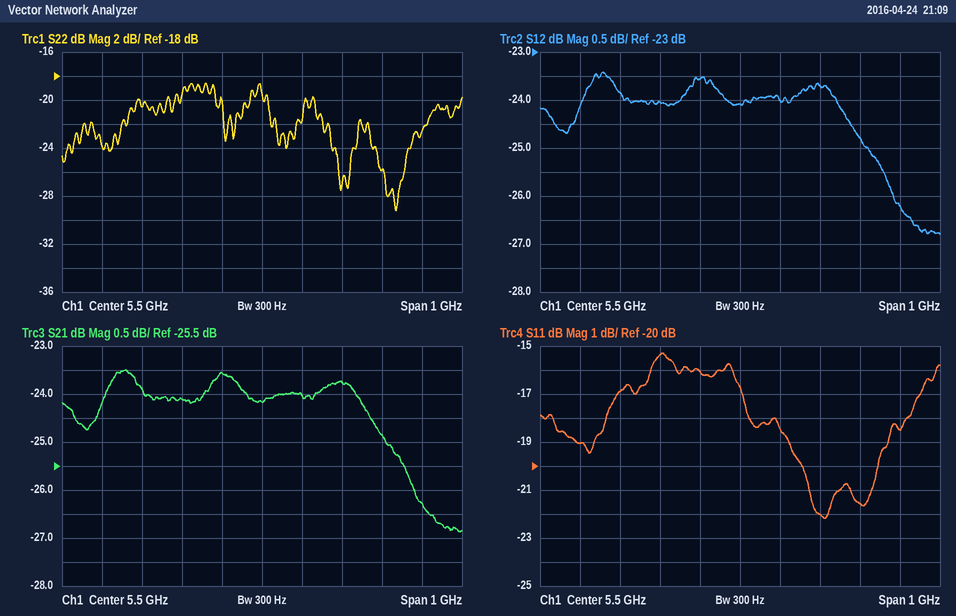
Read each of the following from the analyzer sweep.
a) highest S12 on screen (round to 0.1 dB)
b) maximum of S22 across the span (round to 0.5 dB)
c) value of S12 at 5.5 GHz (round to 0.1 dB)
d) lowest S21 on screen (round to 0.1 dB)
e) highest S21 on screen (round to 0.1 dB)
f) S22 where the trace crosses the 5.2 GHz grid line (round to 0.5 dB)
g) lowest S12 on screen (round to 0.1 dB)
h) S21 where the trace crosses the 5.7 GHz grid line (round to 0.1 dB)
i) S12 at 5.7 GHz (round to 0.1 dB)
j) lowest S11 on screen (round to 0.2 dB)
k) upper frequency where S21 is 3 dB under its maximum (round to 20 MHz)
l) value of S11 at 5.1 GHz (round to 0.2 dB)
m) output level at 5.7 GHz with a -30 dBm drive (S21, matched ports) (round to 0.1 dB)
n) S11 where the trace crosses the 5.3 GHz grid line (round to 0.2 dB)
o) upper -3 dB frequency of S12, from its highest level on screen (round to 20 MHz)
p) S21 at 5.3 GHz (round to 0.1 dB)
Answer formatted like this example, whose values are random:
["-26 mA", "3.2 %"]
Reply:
["-23.4 dB", "-18.5 dB", "-24.1 dB", "-26.9 dB", "-23.5 dB", "-20.5 dB", "-26.8 dB", "-23.8 dB", "-23.7 dB", "-22.2 dB", "5.92 GHz", "-19.0 dB", "-53.8 dBm", "-15.4 dB", "5.92 GHz", "-24.1 dB"]
